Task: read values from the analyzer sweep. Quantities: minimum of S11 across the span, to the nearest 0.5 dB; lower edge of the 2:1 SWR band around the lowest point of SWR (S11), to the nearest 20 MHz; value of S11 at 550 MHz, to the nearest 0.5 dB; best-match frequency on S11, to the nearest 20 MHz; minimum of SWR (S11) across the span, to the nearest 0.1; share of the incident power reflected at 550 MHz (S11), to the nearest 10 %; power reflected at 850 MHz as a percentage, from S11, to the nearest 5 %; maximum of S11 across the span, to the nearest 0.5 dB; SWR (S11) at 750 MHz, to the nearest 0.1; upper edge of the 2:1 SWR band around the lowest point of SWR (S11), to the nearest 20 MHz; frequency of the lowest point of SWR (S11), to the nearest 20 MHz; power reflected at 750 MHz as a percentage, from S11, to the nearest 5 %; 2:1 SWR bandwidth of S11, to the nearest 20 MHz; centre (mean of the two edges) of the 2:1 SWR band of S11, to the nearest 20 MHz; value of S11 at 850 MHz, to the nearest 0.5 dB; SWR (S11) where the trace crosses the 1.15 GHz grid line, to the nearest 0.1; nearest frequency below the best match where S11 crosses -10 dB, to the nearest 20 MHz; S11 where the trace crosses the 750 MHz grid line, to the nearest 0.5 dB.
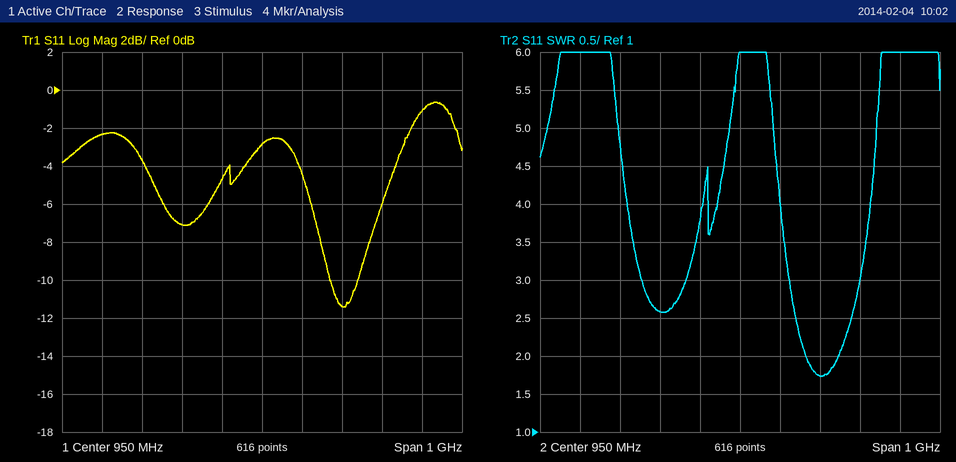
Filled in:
-11.5 dB
1.12 GHz
-2.5 dB
1.16 GHz
1.7
60 %
35 %
-0.5 dB
2.6
1.20 GHz
1.16 GHz
20 %
80 MHz
1.16 GHz
-4.5 dB
1.7
1.12 GHz
-7.0 dB
